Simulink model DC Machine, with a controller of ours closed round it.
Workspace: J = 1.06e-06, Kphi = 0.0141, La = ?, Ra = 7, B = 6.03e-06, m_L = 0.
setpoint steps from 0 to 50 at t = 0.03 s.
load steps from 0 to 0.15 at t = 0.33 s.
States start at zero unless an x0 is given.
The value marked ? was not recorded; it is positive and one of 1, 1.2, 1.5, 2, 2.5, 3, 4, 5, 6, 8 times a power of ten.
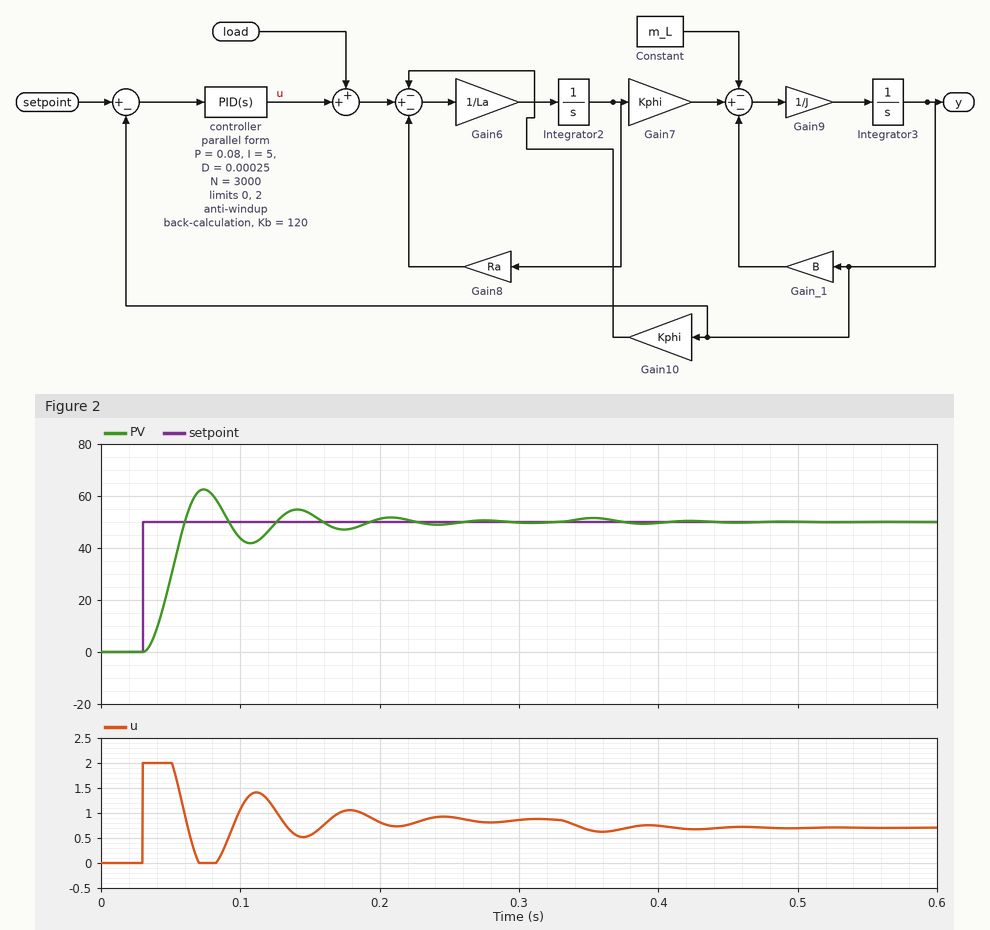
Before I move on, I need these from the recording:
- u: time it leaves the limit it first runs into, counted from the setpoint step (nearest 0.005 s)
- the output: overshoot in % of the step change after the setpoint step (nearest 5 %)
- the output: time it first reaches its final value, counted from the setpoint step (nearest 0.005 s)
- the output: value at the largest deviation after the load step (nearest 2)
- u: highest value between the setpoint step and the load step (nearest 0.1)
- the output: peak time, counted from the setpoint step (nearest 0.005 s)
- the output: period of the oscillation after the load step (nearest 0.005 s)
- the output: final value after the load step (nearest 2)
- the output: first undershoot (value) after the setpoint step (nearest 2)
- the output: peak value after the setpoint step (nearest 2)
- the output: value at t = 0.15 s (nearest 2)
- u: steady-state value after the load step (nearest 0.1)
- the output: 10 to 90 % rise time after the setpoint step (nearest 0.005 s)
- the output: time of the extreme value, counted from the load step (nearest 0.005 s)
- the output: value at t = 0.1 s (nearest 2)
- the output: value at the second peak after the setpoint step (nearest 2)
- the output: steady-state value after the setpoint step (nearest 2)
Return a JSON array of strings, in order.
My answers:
["0.020 s", "25 %", "0.030 s", "52", "2.0", "0.045 s", "0.070 s", "50", "42", "62", "54", "0.7", "0.020 s", "0.025 s", "44", "54", "50"]
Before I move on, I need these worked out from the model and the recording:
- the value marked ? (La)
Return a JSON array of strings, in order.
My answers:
["0.12"]
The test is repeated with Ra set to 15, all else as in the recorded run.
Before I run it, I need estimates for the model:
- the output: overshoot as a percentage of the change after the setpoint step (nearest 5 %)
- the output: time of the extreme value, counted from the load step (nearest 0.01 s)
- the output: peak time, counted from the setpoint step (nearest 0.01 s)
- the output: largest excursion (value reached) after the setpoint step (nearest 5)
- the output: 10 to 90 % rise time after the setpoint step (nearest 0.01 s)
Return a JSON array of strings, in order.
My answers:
["15 %", "0.03 s", "0.06 s", "55", "0.03 s"]
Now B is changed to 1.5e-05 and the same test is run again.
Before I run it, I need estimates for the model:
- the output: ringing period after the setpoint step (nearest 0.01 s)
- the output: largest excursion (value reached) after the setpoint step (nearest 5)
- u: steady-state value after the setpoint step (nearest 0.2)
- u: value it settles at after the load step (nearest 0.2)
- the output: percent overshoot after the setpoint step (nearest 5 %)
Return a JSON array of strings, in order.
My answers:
["0.07 s", "60", "1.0", "1.0", "20 %"]
